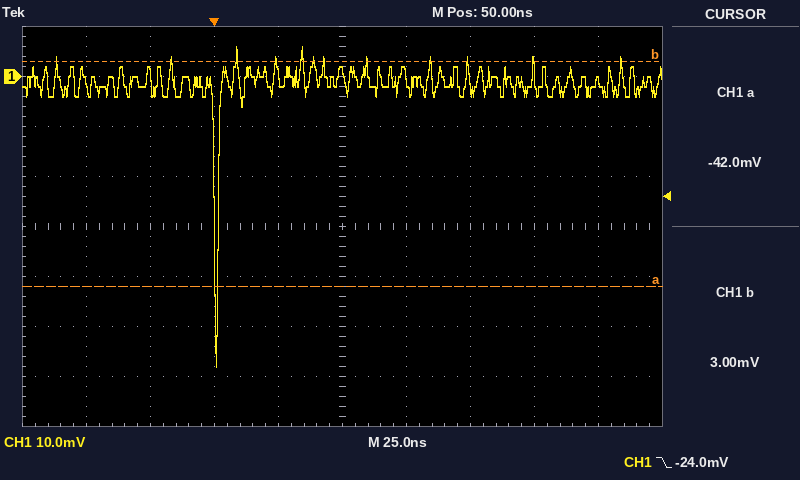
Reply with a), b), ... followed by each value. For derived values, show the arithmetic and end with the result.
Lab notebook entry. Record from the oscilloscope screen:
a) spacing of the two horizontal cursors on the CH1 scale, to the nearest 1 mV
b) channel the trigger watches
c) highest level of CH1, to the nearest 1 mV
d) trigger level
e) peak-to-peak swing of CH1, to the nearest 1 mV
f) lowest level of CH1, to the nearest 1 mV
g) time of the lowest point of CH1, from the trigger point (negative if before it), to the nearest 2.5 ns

a) 45 mV
b) CH1
c) 6 mV
d) -24.0 mV
e) 6 mV − (-58 mV) = 64 mV
f) -58 mV
g) 0.0 ns
